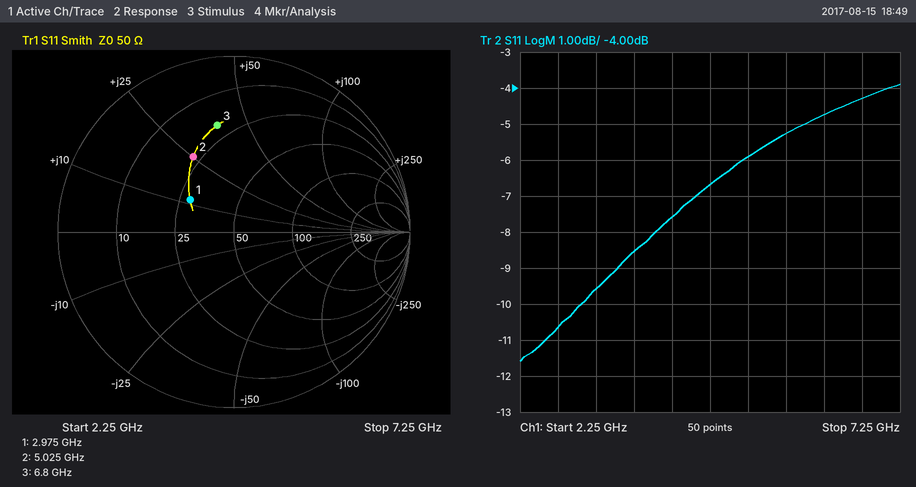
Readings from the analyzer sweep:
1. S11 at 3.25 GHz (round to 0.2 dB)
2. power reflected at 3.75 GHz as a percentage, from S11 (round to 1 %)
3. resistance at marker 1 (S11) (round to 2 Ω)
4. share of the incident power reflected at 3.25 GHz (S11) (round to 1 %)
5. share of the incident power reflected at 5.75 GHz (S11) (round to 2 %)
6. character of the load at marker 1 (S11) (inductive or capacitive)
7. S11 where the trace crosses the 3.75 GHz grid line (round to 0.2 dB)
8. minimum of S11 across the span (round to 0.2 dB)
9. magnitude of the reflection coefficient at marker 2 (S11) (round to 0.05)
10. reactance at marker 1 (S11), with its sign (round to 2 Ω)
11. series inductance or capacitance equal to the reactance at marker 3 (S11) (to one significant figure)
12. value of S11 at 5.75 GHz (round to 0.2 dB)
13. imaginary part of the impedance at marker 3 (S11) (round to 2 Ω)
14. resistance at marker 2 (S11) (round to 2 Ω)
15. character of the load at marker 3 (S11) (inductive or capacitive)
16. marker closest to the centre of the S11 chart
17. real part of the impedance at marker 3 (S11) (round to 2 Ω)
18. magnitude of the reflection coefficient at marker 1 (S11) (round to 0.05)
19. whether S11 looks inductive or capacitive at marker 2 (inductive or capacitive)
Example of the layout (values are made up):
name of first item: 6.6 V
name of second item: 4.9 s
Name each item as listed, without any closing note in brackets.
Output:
S11 at 3.25 GHz: -9.6 dB
power reflected at 3.75 GHz as a percentage, from S11: 14 %
resistance at marker 1 (S11): 28 Ω
share of the incident power reflected at 3.25 GHz (S11): 11 %
share of the incident power reflected at 5.75 GHz (S11): 30 %
character of the load at marker 1 (S11): inductive
S11 where the trace crosses the 3.75 GHz grid line: -8.6 dB
minimum of S11 across the span: -11.6 dB
magnitude of the reflection coefficient at marker 2 (S11): 0.50
reactance at marker 1 (S11), with its sign: +12 Ω
series inductance or capacitance equal to the reactance at marker 3 (S11): 900 pH
value of S11 at 5.75 GHz: -5.2 dB
imaginary part of the impedance at marker 3 (S11): +38 Ω
resistance at marker 2 (S11): 22 Ω
character of the load at marker 3 (S11): inductive
marker closest to the centre of the S11 chart: marker 1
real part of the impedance at marker 3 (S11): 20 Ω
magnitude of the reflection coefficient at marker 1 (S11): 0.30
whether S11 looks inductive or capacitive at marker 2: inductive
